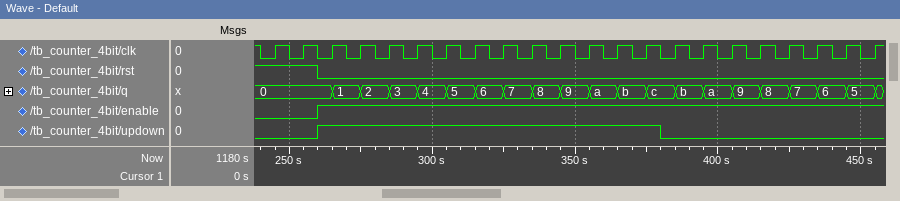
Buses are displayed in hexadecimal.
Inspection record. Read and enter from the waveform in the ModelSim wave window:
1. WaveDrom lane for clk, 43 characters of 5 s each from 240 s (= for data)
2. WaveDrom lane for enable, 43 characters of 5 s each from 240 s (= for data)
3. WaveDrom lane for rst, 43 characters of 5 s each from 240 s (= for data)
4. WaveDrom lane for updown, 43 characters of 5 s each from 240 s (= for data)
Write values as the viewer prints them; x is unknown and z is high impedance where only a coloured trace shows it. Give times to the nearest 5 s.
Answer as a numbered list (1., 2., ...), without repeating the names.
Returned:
1. {name: 'clk', wave: '0101010101010101010101010101010101010101010'}
2. {name: 'enable', wave: '0...1......................................'}
3. {name: 'rst', wave: '1...0......................................'}
4. {name: 'updown', wave: '0...1.......................0..............'}
